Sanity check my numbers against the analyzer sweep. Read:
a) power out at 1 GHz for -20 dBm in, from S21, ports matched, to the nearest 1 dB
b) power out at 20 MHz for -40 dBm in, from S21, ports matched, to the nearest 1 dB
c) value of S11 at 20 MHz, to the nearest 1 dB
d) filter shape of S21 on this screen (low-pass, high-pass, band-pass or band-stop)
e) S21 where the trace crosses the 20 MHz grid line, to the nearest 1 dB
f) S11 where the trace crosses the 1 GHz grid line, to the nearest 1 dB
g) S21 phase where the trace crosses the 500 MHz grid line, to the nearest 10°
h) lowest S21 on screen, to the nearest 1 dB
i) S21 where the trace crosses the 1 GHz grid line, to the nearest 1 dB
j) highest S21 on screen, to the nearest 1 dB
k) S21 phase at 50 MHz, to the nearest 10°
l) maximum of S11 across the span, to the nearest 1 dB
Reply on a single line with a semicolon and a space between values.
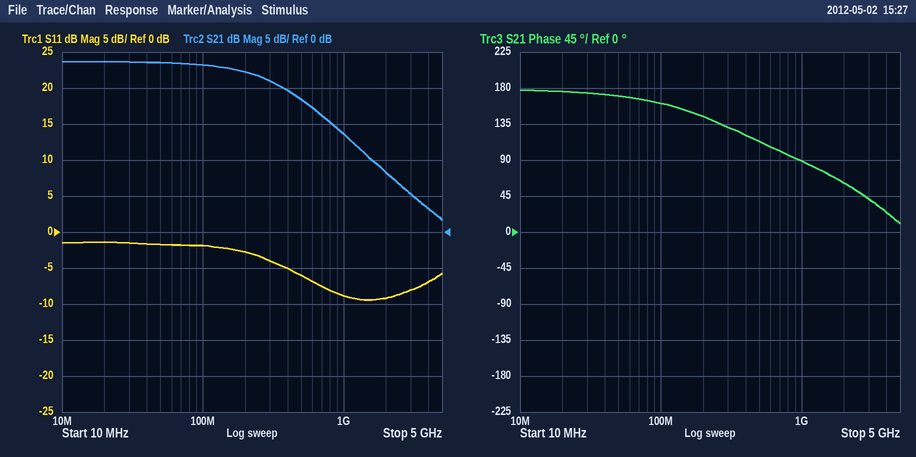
-6 dBm; -16 dBm; -1 dB; low-pass; 24 dB; -9 dB; 110°; 2 dB; 14 dB; 24 dB; 170°; -1 dB
